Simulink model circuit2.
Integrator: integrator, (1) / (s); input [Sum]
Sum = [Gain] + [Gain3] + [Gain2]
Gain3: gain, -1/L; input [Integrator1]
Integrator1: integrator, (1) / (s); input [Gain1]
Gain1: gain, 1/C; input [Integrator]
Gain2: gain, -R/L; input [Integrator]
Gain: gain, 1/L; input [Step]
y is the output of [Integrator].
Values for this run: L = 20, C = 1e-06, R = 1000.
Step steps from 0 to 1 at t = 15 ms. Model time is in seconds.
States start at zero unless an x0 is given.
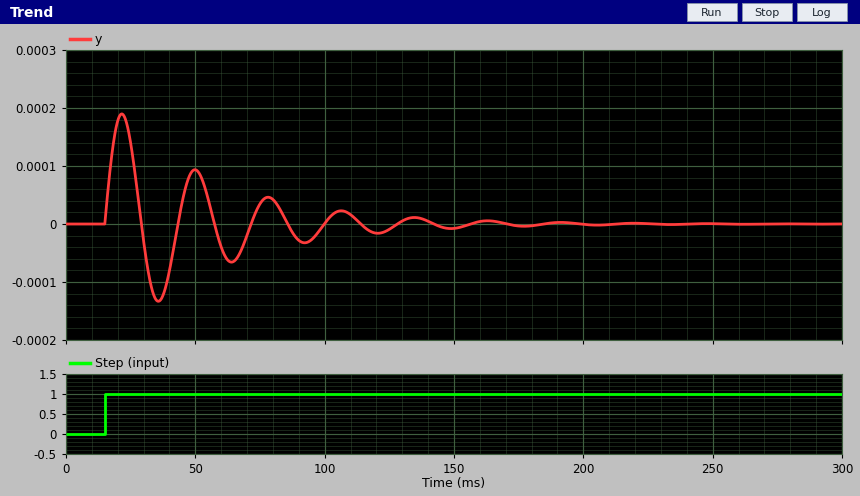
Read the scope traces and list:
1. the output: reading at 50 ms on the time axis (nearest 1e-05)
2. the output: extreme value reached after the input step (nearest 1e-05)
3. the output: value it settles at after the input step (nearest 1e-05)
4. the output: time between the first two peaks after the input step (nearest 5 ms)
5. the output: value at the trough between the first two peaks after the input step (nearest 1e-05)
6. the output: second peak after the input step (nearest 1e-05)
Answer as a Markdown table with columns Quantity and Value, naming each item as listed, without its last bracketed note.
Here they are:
| Quantity | Value |
|---|---|
| the output: reading at 50 ms on the time axis | 0.00009 |
| the output: extreme value reached after the input step | 0.00019 |
| the output: value it settles at after the input step | 0.00000 |
| the output: time between the first two peaks after the input step | 30 ms |
| the output: value at the trough between the first two peaks after the input step | -0.00013 |
| the output: second peak after the input step | 0.00009 |
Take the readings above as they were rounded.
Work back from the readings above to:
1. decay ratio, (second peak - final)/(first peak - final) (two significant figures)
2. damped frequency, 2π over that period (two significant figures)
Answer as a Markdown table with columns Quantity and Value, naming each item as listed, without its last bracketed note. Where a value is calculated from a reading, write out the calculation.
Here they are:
| Quantity | Value |
|---|---|
| decay ratio, (second peak - final)/(first peak - final) | (9e-05 - 0) / (0.00019 - 0) = 0.47 |
| damped frequency, 2π over that period | 2π / 30 = 0.21 rad/ms |
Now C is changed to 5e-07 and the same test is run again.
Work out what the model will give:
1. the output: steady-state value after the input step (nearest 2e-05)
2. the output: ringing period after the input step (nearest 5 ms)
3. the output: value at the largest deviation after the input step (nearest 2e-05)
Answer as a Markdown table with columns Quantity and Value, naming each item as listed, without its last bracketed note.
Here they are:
| Quantity | Value |
|---|---|
| the output: steady-state value after the input step | 0.00000 |
| the output: ringing period after the input step | 20 ms |
| the output: value at the largest deviation after the input step | 0.00014 |
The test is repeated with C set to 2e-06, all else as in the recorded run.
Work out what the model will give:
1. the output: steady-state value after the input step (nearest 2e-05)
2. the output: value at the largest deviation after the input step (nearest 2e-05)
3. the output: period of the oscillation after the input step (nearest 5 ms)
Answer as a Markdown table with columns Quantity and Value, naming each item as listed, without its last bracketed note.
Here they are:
| Quantity | Value |
|---|---|
| the output: steady-state value after the input step | 0.00000 |
| the output: value at the largest deviation after the input step | 0.00026 |
| the output: period of the oscillation after the input step | 40 ms |
